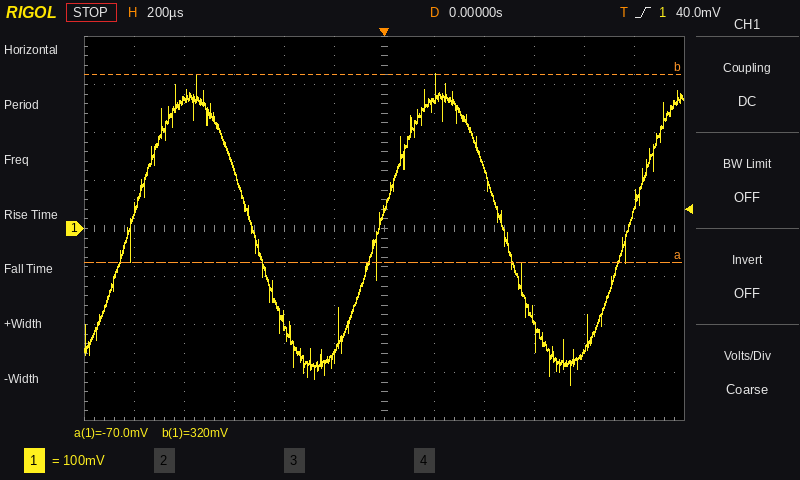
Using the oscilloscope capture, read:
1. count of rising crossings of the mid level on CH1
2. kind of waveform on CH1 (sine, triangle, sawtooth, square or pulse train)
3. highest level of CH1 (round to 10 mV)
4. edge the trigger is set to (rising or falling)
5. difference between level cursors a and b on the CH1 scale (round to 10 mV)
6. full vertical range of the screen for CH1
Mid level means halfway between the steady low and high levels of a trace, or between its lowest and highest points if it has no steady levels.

3
sine
320 mV
rising
390 mV
800 mV
